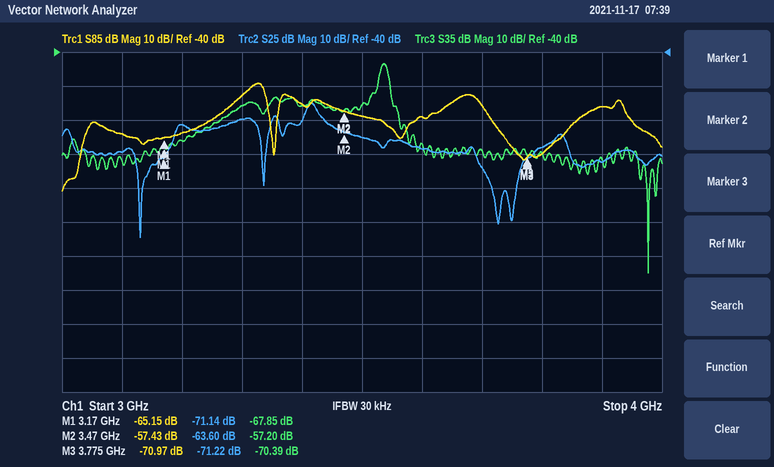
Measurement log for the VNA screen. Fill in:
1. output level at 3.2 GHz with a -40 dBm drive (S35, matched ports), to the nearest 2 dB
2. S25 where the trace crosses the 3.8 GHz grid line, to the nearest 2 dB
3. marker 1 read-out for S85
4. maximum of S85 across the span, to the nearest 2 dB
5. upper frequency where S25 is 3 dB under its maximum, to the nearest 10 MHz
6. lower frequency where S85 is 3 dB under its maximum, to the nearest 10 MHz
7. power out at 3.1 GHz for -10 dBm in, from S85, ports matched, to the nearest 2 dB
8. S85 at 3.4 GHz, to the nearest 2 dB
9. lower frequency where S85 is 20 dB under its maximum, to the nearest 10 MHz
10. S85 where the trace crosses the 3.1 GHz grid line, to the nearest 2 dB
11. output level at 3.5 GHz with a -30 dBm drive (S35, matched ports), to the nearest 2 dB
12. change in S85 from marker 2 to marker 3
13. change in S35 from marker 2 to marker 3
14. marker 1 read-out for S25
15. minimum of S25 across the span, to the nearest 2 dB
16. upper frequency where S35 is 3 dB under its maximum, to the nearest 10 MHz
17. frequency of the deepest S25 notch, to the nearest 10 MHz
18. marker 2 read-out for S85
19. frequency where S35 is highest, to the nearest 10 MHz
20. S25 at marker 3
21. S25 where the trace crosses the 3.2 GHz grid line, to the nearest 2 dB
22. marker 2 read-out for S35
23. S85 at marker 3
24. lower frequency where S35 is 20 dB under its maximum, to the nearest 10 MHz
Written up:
-106 dBm
-68 dB
-65.15 dB
-50 dB
3.43 GHz
3.30 GHz
-74 dBm
-56 dB
3.03 GHz
-64 dB
-86 dBm
-13.54 dB
-13.19 dB
-71.14 dB
-94 dB
3.54 GHz
3.13 GHz
-57.43 dB
3.54 GHz
-71.22 dB
-62 dB
-57.20 dB
-70.97 dB
3.23 GHz
